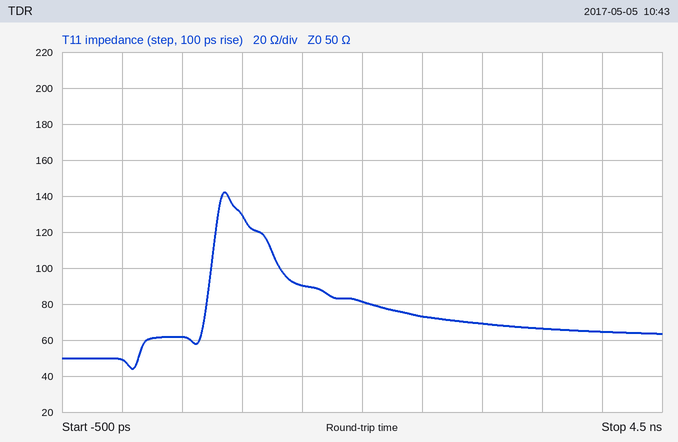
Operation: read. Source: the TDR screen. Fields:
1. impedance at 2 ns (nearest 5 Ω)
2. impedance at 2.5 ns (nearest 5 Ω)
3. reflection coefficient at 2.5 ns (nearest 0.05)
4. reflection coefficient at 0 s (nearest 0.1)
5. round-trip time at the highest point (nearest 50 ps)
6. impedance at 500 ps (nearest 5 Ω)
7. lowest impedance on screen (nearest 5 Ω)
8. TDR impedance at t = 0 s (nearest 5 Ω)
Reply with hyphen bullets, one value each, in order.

- 80 Ω
- 75 Ω
- +0.20
- 0.0
- 850 ps
- 60 Ω
- 45 Ω
- 50 Ω
